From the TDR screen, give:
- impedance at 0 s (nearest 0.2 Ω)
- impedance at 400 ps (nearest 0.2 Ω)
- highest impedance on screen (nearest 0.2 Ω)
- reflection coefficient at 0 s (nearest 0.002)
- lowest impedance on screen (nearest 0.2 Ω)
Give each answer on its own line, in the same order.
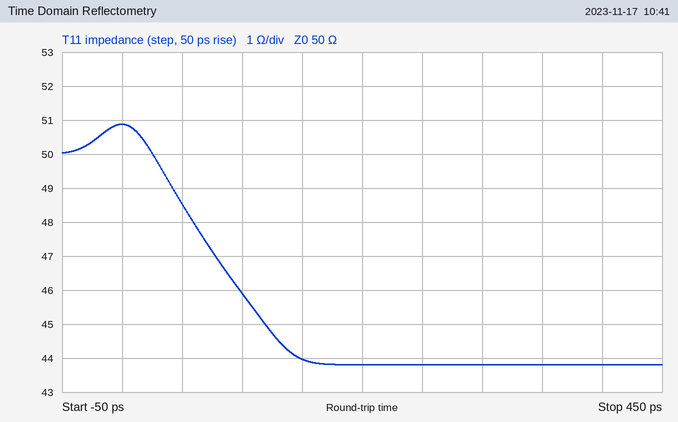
50.8 Ω
43.8 Ω
50.8 Ω
+0.008
43.8 Ω
